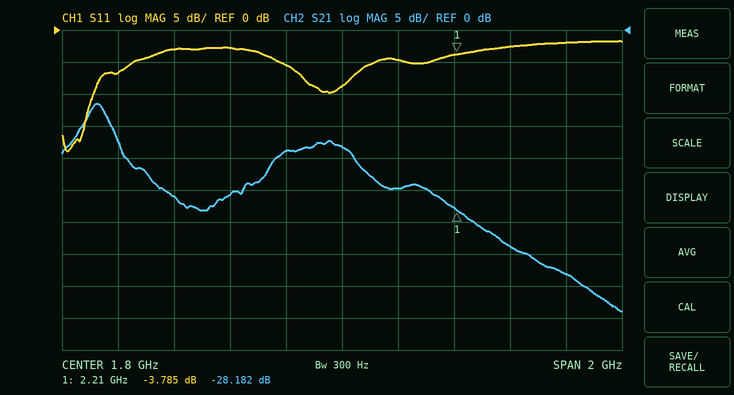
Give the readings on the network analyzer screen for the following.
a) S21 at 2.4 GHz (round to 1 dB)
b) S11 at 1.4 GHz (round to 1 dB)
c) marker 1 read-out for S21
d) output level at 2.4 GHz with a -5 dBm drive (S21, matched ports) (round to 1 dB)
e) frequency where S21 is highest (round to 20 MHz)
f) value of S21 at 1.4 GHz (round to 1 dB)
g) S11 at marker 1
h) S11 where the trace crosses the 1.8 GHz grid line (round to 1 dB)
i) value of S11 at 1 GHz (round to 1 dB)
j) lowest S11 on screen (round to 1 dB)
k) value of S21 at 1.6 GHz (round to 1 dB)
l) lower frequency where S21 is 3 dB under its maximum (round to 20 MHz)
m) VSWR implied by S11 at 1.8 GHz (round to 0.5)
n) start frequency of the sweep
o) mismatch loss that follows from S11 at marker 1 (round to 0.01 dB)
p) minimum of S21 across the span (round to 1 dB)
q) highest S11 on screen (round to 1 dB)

-34 dB
-3 dB
-28.182 dB
-39 dBm
920 MHz
-26 dB
-3.785 dB
-9 dB
-7 dB
-19 dB
-19 dB
880 MHz
2.0
800 MHz
2.35 dB
-44 dB
-2 dB
